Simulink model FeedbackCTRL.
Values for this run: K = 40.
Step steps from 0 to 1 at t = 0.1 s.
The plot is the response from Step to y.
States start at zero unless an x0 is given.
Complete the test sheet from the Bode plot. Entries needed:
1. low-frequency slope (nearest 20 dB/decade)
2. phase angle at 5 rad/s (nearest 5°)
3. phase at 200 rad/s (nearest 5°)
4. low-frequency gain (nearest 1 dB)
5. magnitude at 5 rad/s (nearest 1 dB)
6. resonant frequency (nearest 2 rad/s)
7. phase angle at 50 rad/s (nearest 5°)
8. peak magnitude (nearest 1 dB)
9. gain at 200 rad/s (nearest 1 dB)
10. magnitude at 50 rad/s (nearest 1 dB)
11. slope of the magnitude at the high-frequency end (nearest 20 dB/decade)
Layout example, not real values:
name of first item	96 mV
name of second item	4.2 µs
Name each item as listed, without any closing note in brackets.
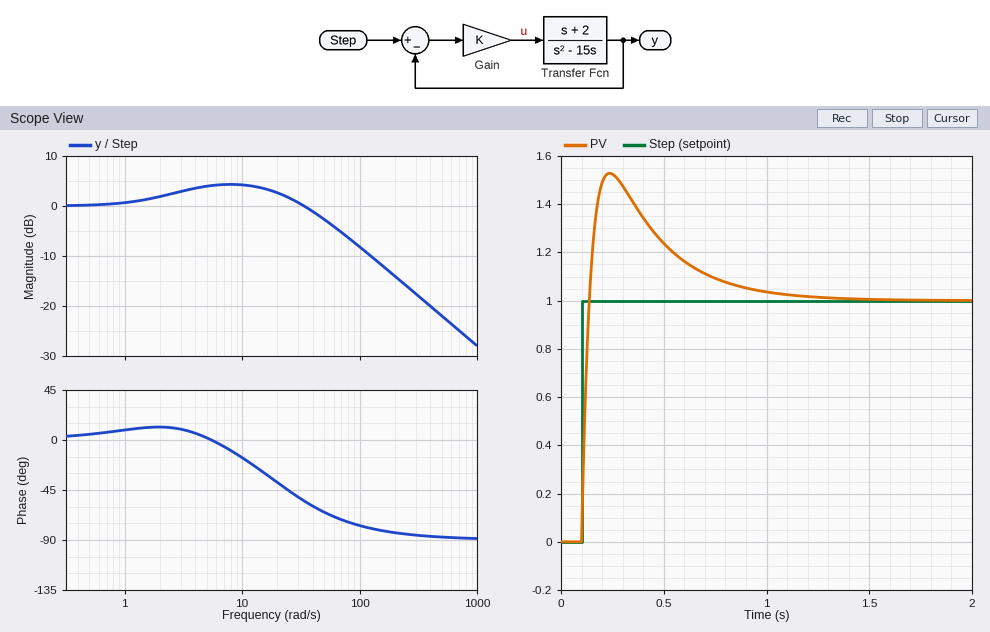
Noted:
low-frequency slope	0 dB/decade
phase angle at 5 rad/s	0°
phase at 200 rad/s	-85°
low-frequency gain	0 dB
magnitude at 5 rad/s	4 dB
resonant frequency	8 rad/s
phase angle at 50 rad/s	-65°
peak magnitude	4 dB
gain at 200 rad/s	-14 dB
magnitude at 50 rad/s	-3 dB
slope of the magnitude at the high-frequency end	-20 dB/decade
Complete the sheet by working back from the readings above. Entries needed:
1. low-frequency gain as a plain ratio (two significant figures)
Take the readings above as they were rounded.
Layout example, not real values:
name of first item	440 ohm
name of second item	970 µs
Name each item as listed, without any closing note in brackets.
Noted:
low-frequency gain as a plain ratio	1.0
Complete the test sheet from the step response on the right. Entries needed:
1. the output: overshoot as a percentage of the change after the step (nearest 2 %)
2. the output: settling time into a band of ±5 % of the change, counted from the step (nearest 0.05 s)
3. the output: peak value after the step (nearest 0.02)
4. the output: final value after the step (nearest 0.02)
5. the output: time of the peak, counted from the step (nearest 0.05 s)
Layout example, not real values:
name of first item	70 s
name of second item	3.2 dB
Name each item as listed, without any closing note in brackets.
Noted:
the output: overshoot as a percentage of the change after the step	52 %
the output: settling time into a band of ±5 % of the change, counted from the step	0.80 s
the output: peak value after the step	1.52
the output: final value after the step	1.00
the output: time of the peak, counted from the step	0.15 s
